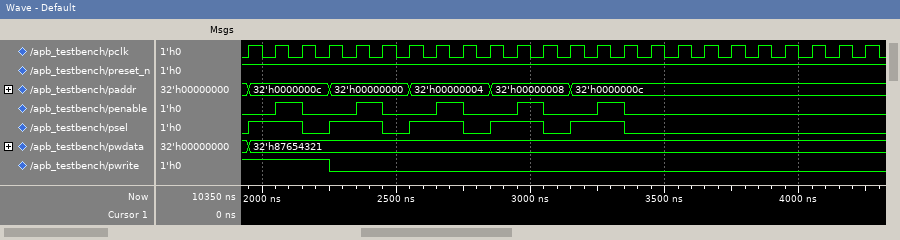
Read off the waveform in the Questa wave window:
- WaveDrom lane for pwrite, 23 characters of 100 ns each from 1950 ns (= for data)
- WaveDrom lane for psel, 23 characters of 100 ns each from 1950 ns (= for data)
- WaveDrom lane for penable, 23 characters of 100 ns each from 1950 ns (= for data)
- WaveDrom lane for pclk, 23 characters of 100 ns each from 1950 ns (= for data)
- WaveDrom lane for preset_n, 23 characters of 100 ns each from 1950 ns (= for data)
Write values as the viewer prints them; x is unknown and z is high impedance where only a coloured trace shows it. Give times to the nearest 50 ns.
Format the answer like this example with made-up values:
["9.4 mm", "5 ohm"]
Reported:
["{name: 'pwrite', wave: '1..0...................'}", "{name: 'psel', wave: '1.01.01.01.01.0........'}", "{name: 'penable', wave: '010.10.10.10.10........'}", "{name: 'pclk', wave: 'p......................'}", "{name: 'preset_n', wave: '1......................'}"]
